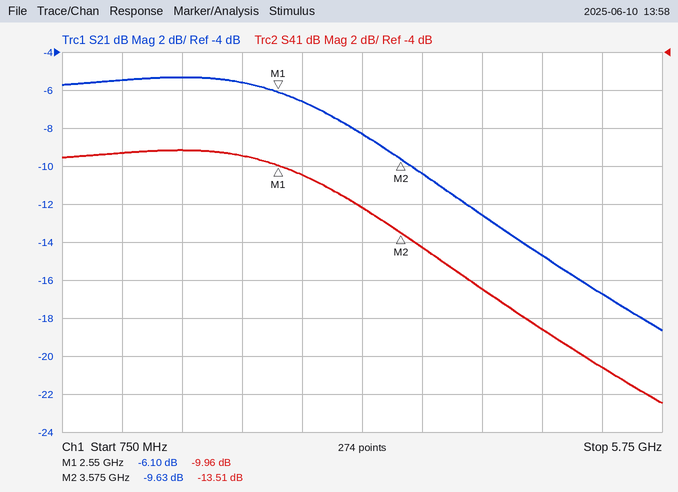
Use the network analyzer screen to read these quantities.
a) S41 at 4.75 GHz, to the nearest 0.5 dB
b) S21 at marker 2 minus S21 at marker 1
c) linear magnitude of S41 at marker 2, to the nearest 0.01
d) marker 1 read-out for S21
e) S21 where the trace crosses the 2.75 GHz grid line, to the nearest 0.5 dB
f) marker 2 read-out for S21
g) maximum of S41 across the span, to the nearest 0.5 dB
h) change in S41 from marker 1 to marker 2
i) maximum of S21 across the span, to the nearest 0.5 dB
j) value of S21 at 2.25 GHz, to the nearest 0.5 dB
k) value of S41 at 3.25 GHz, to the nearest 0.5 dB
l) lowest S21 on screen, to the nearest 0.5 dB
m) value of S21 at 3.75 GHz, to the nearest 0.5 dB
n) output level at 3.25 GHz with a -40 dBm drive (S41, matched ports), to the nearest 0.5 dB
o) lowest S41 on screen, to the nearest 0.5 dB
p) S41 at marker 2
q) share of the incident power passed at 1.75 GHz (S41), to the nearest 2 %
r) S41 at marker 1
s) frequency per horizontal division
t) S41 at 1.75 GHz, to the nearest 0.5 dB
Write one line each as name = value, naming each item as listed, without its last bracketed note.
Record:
S41 at 4.75 GHz, to the nearest 0.5 dB = -18.5 dB
S21 at marker 2 minus S21 at marker 1 = -3.53 dB
linear magnitude of S41 at marker 2, to the nearest 0.01 = 0.21
marker 1 read-out for S21 = -6.10 dB
S21 where the trace crosses the 2.75 GHz grid line, to the nearest 0.5 dB = -6.5 dB
marker 2 read-out for S21 = -9.63 dB
maximum of S41 across the span, to the nearest 0.5 dB = -9.0 dB
change in S41 from marker 1 to marker 2 = -3.55 dB
maximum of S21 across the span, to the nearest 0.5 dB = -5.5 dB
value of S21 at 2.25 GHz, to the nearest 0.5 dB = -5.5 dB
value of S41 at 3.25 GHz, to the nearest 0.5 dB = -12.0 dB
lowest S21 on screen, to the nearest 0.5 dB = -18.5 dB
value of S21 at 3.75 GHz, to the nearest 0.5 dB = -10.5 dB
output level at 3.25 GHz with a -40 dBm drive (S41, matched ports), to the nearest 0.5 dB = -52.0 dBm
lowest S41 on screen, to the nearest 0.5 dB = -22.5 dB
S41 at marker 2 = -13.51 dB
share of the incident power passed at 1.75 GHz (S41), to the nearest 2 % = 12 %
S41 at marker 1 = -9.96 dB
frequency per horizontal division = 500 MHz
S41 at 1.75 GHz, to the nearest 0.5 dB = -9.0 dB
